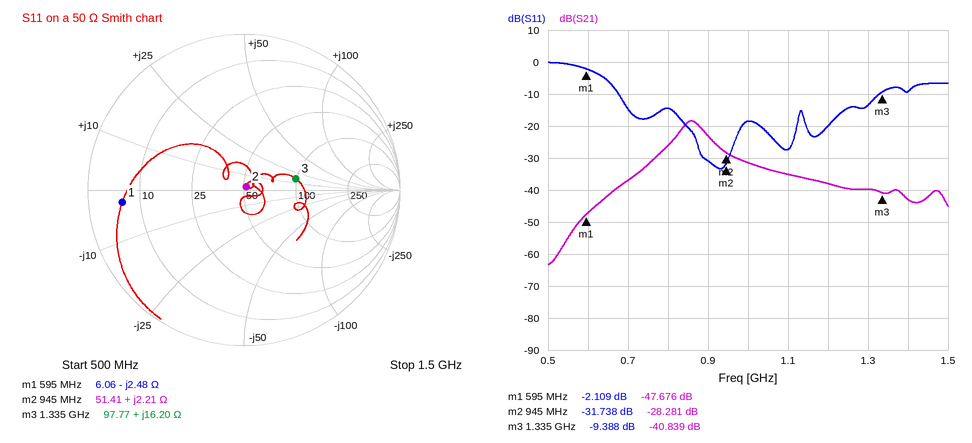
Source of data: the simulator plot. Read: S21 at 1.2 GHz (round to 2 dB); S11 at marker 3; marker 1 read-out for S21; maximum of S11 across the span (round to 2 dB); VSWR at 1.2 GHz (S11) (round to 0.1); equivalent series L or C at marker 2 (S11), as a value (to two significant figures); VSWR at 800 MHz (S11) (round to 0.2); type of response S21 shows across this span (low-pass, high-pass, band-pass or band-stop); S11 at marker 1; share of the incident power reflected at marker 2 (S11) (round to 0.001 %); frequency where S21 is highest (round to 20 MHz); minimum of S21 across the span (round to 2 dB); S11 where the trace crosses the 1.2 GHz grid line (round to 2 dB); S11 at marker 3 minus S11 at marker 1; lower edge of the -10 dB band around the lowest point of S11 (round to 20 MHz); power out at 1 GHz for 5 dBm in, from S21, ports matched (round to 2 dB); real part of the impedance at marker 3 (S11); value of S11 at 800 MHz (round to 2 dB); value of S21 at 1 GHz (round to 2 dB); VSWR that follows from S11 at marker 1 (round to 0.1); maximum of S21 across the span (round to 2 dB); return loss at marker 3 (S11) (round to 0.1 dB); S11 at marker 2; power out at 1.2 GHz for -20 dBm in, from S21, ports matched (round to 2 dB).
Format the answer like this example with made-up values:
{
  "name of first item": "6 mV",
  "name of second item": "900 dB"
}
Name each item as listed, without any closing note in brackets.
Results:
{
  "S21 at 1.2 GHz": "-38 dB",
  "S11 at marker 3": "-9.388 dB",
  "marker 1 read-out for S21": "-47.676 dB",
  "maximum of S11 across the span": "0 dB",
  "VSWR at 1.2 GHz (S11)": "1.2",
  "equivalent series L or C at marker 2 (S11), as a value": "370 pH",
  "VSWR at 800 MHz (S11)": "1.4",
  "type of response S21 shows across this span": "band-pass",
  "S11 at marker 1": "-2.109 dB",
  "share of the incident power reflected at marker 2 (S11)": "0.067 %",
  "frequency where S21 is highest": "860 MHz",
  "minimum of S21 across the span": "-64 dB",
  "S11 where the trace crosses the 1.2 GHz grid line": "-20 dB",
  "S11 at marker 3 minus S11 at marker 1": "-7.279 dB",
  "lower edge of the -10 dB band around the lowest point of S11": "680 MHz",
  "power out at 1 GHz for 5 dBm in, from S21, ports matched": "-26 dBm",
  "real part of the impedance at marker 3": "97.77 Ω",
  "value of S11 at 800 MHz": "-14 dB",
  "value of S21 at 1 GHz": "-32 dB",
  "VSWR that follows from S11 at marker 1": "8.3",
  "maximum of S21 across the span": "-18 dB",
  "return loss at marker 3 (S11)": "9.4 dB",
  "S11 at marker 2": "-31.738 dB",
  "power out at 1.2 GHz for -20 dBm in, from S21, ports matched": "-58 dBm"
}
